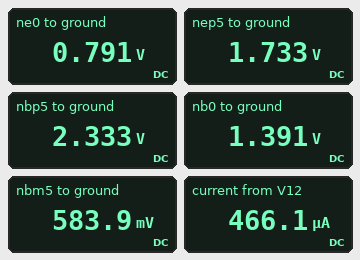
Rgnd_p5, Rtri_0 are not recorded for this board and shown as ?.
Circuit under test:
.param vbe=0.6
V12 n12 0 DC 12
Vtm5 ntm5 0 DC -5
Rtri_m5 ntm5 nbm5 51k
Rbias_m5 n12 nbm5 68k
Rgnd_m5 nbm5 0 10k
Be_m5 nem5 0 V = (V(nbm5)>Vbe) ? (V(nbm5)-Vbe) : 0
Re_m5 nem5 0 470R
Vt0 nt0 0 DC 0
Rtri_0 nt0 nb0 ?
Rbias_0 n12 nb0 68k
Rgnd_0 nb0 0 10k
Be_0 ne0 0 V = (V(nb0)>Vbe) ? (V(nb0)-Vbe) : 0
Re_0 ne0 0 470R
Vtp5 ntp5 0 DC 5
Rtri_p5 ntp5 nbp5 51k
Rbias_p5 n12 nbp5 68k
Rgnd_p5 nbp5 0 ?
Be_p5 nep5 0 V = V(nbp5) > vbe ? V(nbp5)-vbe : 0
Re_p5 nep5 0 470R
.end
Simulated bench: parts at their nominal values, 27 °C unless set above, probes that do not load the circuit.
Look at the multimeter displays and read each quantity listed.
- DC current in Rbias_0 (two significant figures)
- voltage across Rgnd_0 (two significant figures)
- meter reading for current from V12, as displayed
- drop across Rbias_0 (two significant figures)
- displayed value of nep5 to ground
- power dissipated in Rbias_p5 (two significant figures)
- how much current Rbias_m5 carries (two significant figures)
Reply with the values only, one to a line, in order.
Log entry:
160 µA
1.4 V
466.1 µA
11 V
1.733 V
1.4 mW
170 µA
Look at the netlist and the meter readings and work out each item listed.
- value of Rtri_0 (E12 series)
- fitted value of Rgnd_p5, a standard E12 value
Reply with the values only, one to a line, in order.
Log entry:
82 kΩ
12 kΩ
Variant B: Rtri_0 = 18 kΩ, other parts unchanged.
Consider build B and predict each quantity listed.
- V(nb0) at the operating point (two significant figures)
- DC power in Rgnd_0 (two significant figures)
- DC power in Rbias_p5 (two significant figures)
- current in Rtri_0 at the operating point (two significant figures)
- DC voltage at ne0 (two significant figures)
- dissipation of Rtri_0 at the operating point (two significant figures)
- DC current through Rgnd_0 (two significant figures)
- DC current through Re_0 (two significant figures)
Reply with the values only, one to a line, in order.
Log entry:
1.0 V
110 µW
1.4 mW
58 µA
440 mV
60 µW
100 µA
930 µA
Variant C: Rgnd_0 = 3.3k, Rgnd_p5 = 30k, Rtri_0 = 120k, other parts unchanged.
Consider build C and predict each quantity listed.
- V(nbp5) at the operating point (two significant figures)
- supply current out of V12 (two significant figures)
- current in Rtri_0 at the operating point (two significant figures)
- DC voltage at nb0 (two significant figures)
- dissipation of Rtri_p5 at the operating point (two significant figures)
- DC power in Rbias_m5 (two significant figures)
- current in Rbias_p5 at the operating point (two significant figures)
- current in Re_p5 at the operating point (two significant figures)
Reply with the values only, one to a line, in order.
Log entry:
4.1 V
450 µA
4.5 µA
540 mV
17 µW
1.9 mW
120 µA
7.4 mA
